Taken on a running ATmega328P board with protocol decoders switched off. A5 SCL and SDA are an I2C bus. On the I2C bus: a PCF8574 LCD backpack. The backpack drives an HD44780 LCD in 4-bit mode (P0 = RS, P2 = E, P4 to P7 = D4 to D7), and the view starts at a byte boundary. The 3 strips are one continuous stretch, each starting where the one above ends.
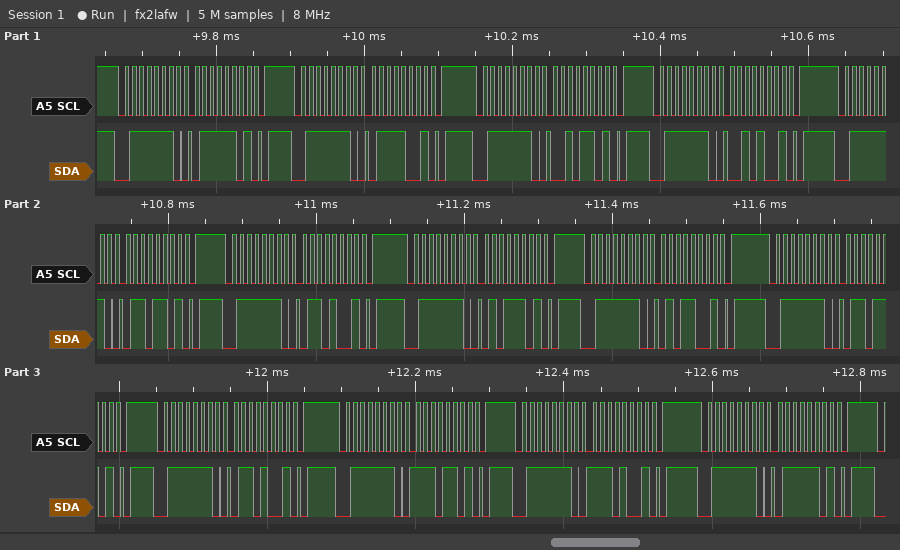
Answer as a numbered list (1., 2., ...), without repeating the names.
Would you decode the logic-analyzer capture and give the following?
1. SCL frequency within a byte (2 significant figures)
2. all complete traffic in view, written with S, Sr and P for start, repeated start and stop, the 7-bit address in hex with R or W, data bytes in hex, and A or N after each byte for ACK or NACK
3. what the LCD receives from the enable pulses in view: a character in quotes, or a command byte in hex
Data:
1. 100 kHz
2. S 3FW A 7D A P S 3FW A 79 A P S 3FW A 2D A P S 3FW A 29 A P S 3FW A 6D A P S 3FW A 69 A P S 3FW A 5D A P S 3FW A 59 A P S 3FW A 6D A P S 3FW A 69 A P S 3FW A ED A P S 3FW A E9 A P S 3FW A 7D A P
3. 'r' 'e' 'n'
